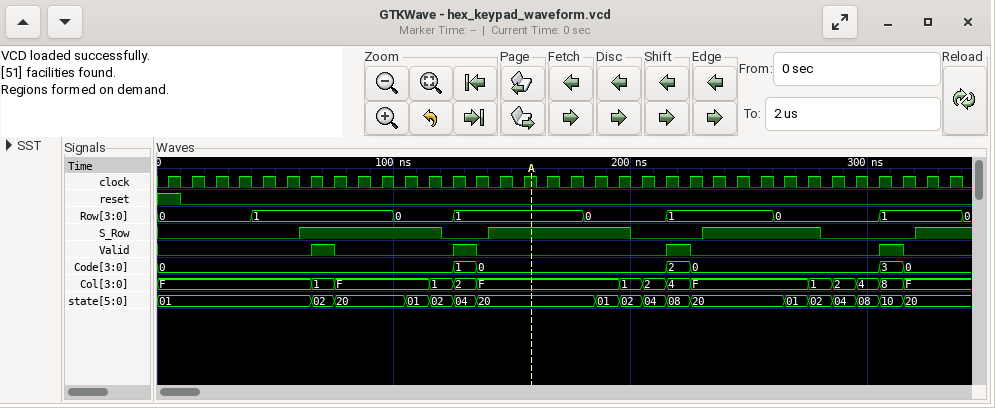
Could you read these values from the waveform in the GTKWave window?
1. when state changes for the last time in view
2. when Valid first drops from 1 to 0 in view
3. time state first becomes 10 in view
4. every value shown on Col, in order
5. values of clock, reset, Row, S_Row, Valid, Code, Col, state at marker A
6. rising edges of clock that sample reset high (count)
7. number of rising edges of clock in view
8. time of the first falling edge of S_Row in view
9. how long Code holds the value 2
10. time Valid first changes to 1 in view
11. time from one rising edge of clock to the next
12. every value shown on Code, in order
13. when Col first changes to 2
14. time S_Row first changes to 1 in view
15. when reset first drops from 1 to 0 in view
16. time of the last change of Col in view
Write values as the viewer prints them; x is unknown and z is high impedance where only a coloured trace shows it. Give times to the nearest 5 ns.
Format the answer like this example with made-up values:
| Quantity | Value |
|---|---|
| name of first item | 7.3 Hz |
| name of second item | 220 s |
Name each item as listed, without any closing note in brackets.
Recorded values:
| Quantity | Value |
|---|---|
| when state changes for the last time in view | 315 ns |
| when Valid first drops from 1 to 0 in view | 75 ns |
| time state first becomes 10 in view | 305 ns |
| every value shown on Col, in order | F, 1, F, 1, 2, F, 1, 2, 4, F, 1, 2, 4, 8, F |
| values of clock, reset, Row, S_Row, Valid, Code, Col, state at marker A | clock=1, reset=0, Row=1, S_Row=1, Valid=0, Code=0, Col=F, state=20 |
| rising edges of clock that sample reset high | 1 |
| number of rising edges of clock in view | 34 |
| time of the first falling edge of S_Row in view | 120 ns |
| how long Code holds the value 2 | 10 ns |
| time Valid first changes to 1 in view | 65 ns |
| time from one rising edge of clock to the next | 10 ns |
| every value shown on Code, in order | 0, 1, 0, 2, 0, 3, 0 |
| when Col first changes to 2 | 125 ns |
| time S_Row first changes to 1 in view | 60 ns |
| when reset first drops from 1 to 0 in view | 10 ns |
| time of the last change of Col in view | 315 ns |
